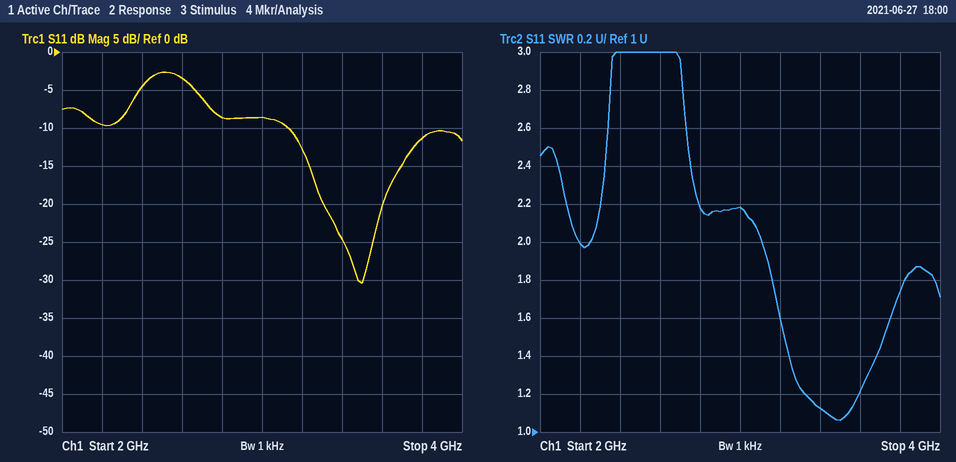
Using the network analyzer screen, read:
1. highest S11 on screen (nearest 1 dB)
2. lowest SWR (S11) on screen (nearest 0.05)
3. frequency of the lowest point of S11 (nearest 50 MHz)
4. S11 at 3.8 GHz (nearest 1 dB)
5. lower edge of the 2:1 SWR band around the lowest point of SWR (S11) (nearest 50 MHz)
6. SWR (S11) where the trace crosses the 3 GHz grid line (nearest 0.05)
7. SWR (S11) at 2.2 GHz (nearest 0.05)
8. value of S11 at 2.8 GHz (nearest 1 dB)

-3 dB
1.05
3.50 GHz
-11 dB
3.10 GHz
2.20
2.00
-9 dB
